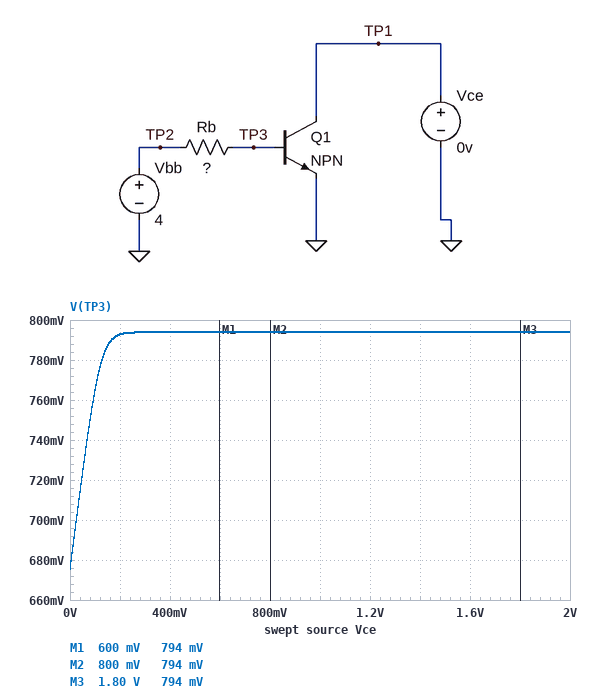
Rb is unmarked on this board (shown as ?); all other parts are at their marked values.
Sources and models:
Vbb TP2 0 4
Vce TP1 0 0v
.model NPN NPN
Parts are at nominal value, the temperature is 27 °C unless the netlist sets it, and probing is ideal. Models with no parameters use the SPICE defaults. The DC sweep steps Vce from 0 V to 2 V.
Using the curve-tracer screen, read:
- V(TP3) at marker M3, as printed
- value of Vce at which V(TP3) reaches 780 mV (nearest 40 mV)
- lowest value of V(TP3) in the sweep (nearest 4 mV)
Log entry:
794 mV
120 mV
676 mV
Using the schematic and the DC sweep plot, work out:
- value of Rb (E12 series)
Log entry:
150 kΩ
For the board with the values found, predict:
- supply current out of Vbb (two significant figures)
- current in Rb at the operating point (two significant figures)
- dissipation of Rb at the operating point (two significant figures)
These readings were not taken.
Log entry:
22 µA
22 µA
74 µW
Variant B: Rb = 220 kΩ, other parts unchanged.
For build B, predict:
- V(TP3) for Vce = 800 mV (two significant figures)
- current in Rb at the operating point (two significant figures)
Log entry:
780 mV
15 µA
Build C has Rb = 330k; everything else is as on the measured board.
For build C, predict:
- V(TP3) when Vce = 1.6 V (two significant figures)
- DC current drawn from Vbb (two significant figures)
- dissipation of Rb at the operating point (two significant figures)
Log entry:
770 mV
10 µA
34 µW
